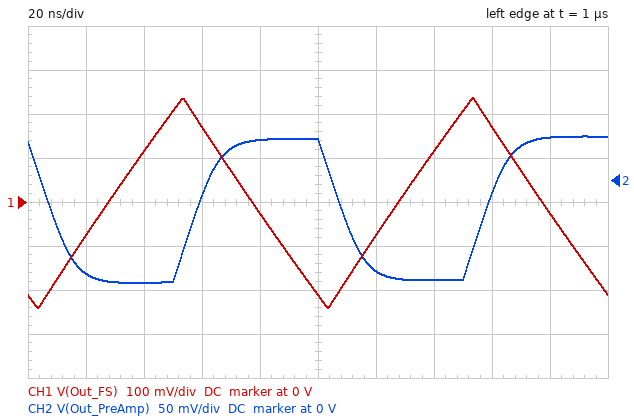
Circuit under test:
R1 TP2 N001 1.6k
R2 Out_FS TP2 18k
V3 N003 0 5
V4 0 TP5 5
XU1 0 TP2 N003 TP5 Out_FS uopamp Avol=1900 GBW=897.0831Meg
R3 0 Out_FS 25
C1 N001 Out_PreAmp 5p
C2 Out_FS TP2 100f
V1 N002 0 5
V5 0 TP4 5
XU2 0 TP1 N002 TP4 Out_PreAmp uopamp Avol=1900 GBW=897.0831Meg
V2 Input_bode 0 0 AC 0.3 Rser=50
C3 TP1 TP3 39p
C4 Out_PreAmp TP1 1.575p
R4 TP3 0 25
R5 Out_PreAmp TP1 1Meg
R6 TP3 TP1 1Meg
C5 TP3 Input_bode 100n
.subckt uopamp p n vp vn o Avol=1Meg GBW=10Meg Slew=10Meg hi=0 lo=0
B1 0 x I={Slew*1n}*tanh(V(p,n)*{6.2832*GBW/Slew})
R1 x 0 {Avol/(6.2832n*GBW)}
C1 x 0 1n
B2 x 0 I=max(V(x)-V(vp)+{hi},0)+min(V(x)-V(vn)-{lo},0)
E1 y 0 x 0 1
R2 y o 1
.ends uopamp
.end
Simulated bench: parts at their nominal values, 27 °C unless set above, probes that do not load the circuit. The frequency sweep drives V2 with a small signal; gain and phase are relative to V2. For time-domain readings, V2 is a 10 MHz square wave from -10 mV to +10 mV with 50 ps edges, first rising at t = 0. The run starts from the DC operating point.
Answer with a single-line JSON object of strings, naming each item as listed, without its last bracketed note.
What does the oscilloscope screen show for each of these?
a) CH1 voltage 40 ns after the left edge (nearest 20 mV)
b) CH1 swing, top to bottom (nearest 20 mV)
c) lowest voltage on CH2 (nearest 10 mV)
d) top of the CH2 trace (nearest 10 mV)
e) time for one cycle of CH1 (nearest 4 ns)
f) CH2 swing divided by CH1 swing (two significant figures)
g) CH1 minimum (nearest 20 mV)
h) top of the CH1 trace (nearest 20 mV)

{"CH1 voltage 40 ns after the left edge": "120 mV", "CH1 swing, top to bottom": "480 mV", "lowest voltage on CH2": "-120 mV", "top of the CH2 trace": "50 mV", "time for one cycle of CH1": "100 ns", "CH2 swing divided by CH1 swing": "0.35", "CH1 minimum": "-240 mV", "top of the CH1 trace": "240 mV"}
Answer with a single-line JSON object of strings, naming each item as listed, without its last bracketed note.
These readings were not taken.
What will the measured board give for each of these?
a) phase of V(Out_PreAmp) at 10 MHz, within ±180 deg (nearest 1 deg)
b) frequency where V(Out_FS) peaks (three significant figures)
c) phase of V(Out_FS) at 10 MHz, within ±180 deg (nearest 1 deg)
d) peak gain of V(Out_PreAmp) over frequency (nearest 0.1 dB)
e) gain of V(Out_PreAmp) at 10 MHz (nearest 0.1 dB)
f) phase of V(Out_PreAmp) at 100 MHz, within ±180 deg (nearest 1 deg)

{"phase of V(Out_PreAmp) at 10 MHz, within ±180 deg": "163 deg", "frequency where V(Out_FS) peaks": "21.6 MHz", "phase of V(Out_FS) at 10 MHz, within ±180 deg": "37 deg", "peak gain of V(Out_PreAmp) over frequency": "18.2 dB", "gain of V(Out_PreAmp) at 10 MHz": "17.8 dB", "phase of V(Out_PreAmp) at 100 MHz, within ±180 deg": "106 deg"}
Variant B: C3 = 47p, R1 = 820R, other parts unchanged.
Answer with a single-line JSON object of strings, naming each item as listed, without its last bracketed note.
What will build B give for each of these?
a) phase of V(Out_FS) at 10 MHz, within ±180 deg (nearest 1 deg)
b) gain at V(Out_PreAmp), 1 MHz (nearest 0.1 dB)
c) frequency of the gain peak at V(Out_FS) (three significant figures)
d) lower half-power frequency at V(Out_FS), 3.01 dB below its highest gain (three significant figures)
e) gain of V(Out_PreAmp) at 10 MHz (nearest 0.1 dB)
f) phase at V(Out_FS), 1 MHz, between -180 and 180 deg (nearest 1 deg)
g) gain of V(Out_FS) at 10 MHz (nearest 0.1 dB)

{"phase of V(Out_FS) at 10 MHz, within ±180 deg": "46 deg", "gain at V(Out_PreAmp), 1 MHz": "19.8 dB", "frequency of the gain peak at V(Out_FS)": "26.1 MHz", "lower half-power frequency at V(Out_FS), 3.01 dB below its highest gain": "13.5 MHz", "gain of V(Out_PreAmp) at 10 MHz": "19.2 dB", "phase at V(Out_FS), 1 MHz, between -180 and 180 deg": "92 deg", "gain of V(Out_FS) at 10 MHz": "34.5 dB"}
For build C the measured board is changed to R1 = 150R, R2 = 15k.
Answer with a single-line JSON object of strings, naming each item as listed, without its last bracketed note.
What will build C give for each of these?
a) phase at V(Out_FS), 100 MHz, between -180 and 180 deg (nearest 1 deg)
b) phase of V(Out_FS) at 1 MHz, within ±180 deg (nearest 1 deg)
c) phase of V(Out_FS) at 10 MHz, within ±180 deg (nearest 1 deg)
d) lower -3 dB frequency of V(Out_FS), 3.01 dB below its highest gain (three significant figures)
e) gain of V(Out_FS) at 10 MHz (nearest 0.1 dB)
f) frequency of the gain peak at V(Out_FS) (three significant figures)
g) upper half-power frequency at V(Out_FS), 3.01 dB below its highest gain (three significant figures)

{"phase at V(Out_FS), 100 MHz, between -180 and 180 deg": "-147 deg", "phase of V(Out_FS) at 1 MHz, within ±180 deg": "94 deg", "phase of V(Out_FS) at 10 MHz, within ±180 deg": "63 deg", "lower -3 dB frequency of V(Out_FS), 3.01 dB below its highest gain": "26.3 MHz", "gain of V(Out_FS) at 10 MHz": "31.7 dB", "frequency of the gain peak at V(Out_FS)": "38.2 MHz", "upper half-power frequency at V(Out_FS), 3.01 dB below its highest gain": "50.1 MHz"}
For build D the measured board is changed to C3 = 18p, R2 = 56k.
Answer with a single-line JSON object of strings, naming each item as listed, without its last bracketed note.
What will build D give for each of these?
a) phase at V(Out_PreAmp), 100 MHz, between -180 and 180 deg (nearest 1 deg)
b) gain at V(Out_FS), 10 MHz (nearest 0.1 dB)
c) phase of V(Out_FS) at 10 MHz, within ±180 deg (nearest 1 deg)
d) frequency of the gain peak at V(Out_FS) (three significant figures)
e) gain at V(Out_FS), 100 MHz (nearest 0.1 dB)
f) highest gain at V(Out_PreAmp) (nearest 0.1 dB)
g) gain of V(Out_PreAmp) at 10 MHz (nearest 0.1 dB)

{"phase at V(Out_PreAmp), 100 MHz, between -180 and 180 deg": "122 deg", "gain at V(Out_FS), 10 MHz": "35.8 dB", "phase of V(Out_FS) at 10 MHz, within ±180 deg": "27 deg", "frequency of the gain peak at V(Out_FS)": "15.7 MHz", "gain at V(Out_FS), 100 MHz": "19.4 dB", "highest gain at V(Out_PreAmp)": "11.6 dB", "gain of V(Out_PreAmp) at 10 MHz": "11.5 dB"}
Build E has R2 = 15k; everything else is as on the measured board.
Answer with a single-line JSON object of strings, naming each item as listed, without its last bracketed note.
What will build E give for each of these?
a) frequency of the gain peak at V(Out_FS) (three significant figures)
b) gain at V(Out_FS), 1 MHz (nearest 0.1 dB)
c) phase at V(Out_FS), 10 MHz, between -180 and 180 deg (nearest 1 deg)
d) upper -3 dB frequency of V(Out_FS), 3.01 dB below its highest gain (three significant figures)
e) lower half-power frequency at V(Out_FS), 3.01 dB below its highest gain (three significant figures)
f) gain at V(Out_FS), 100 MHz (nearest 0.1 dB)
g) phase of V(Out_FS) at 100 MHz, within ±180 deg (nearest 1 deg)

{"frequency of the gain peak at V(Out_FS)": "22.5 MHz", "gain at V(Out_FS), 1 MHz": "11.6 dB", "phase at V(Out_FS), 10 MHz, between -180 and 180 deg": "38 deg", "upper -3 dB frequency of V(Out_FS), 3.01 dB below its highest gain": "43.5 MHz", "lower half-power frequency at V(Out_FS), 3.01 dB below its highest gain": "10.2 MHz", "gain at V(Out_FS), 100 MHz": "20.0 dB", "phase of V(Out_FS) at 100 MHz, within ±180 deg": "-134 deg"}
